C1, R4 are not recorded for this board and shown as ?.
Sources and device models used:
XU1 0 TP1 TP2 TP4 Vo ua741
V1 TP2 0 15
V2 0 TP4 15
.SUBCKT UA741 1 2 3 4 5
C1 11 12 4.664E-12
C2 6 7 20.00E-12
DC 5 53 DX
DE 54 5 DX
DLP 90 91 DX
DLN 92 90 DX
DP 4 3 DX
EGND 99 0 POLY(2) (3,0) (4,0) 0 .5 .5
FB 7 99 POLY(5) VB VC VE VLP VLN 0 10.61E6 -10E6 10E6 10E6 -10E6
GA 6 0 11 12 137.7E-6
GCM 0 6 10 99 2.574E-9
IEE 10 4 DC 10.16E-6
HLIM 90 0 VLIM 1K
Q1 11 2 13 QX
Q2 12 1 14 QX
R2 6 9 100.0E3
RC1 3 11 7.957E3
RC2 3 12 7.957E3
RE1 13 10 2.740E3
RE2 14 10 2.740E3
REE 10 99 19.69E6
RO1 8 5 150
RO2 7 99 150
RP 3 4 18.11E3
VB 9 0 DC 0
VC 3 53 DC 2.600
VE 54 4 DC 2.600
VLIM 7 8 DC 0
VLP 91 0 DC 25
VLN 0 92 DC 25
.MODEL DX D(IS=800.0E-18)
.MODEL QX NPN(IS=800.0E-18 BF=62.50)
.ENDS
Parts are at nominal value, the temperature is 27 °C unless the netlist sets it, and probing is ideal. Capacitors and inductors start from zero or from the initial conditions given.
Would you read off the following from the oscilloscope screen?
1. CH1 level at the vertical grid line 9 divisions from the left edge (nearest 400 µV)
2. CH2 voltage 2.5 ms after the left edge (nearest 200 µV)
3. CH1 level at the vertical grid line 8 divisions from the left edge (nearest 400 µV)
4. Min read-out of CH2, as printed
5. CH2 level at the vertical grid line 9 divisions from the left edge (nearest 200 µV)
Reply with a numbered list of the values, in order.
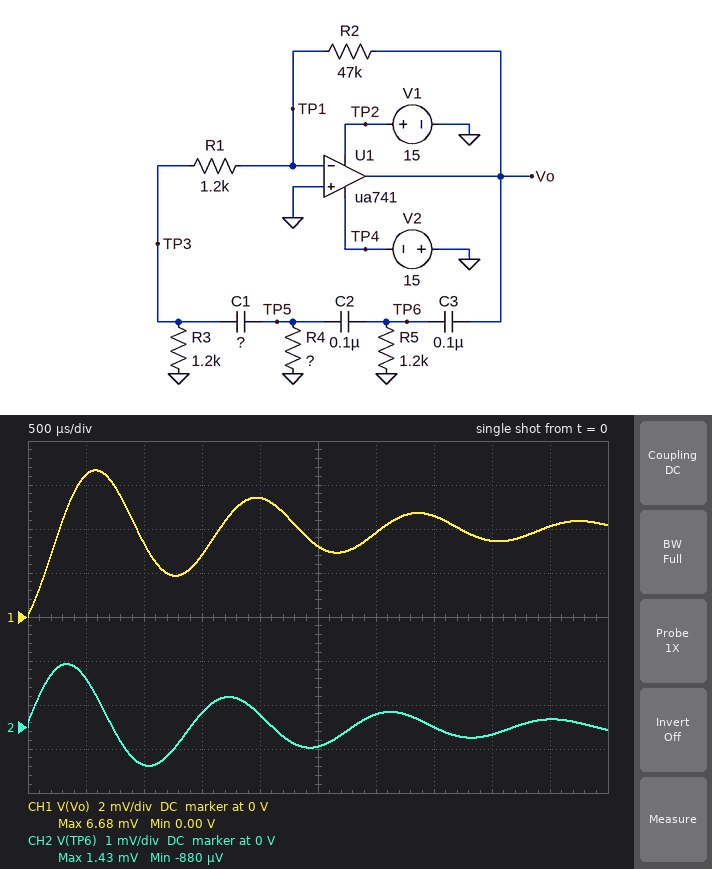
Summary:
1. 4.0 mV
2. -400 µV
3. 3.6 mV
4. -880 µV
5. 200 µV
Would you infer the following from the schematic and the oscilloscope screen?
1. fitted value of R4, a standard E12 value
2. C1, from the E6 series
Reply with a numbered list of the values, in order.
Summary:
1. 3.3 kΩ
2. 33 nF
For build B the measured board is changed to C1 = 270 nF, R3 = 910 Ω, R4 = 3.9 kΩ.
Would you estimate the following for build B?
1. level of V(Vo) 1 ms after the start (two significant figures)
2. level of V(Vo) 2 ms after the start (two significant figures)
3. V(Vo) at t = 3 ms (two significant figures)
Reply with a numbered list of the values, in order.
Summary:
1. 6.4 mV
2. 2.9 mV
3. 4.0 mV
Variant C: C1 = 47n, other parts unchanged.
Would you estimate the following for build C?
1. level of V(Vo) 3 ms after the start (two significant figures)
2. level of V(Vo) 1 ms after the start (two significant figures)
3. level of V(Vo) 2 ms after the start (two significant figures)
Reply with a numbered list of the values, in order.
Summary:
1. 2.7 mV
2. 4.7 mV
3. 4.8 mV
